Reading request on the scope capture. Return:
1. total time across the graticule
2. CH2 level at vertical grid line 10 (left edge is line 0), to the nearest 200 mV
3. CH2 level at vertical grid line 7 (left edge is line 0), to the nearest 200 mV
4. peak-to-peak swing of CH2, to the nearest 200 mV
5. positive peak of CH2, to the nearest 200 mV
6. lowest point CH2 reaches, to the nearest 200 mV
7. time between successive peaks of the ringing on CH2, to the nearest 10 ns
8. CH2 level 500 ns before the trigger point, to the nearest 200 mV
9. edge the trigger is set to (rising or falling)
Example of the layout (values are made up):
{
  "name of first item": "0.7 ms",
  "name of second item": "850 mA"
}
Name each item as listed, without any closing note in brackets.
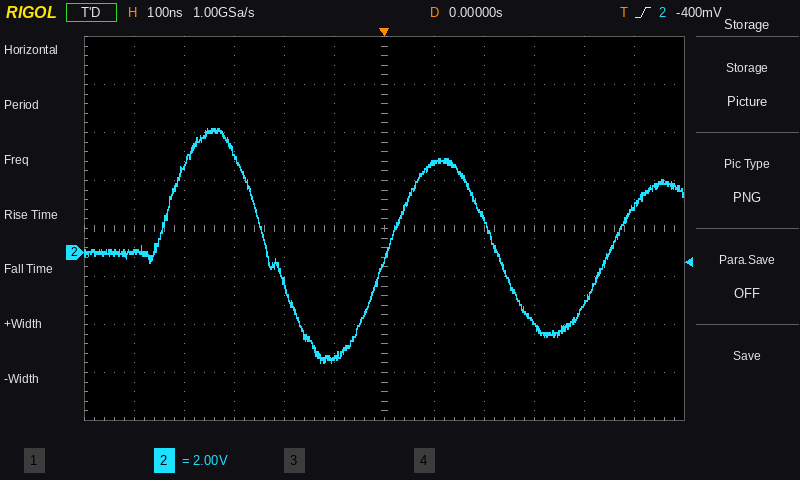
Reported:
{
  "total time across the graticule": "1.2 µs",
  "CH2 level at vertical grid line 10 (left edge is line 0), to the nearest 200 mV": "-2.2 V",
  "CH2 level at vertical grid line 7 (left edge is line 0), to the nearest 200 mV": "3.8 V",
  "peak-to-peak swing of CH2, to the nearest 200 mV": "9.8 V",
  "positive peak of CH2, to the nearest 200 mV": "5.2 V",
  "lowest point CH2 reaches, to the nearest 200 mV": "-4.6 V",
  "time between successive peaks of the ringing on CH2, to the nearest 10 ns": "450 ns",
  "CH2 level 500 ns before the trigger point, to the nearest 200 mV": "0.0 V",
  "edge the trigger is set to": "rising"
}
